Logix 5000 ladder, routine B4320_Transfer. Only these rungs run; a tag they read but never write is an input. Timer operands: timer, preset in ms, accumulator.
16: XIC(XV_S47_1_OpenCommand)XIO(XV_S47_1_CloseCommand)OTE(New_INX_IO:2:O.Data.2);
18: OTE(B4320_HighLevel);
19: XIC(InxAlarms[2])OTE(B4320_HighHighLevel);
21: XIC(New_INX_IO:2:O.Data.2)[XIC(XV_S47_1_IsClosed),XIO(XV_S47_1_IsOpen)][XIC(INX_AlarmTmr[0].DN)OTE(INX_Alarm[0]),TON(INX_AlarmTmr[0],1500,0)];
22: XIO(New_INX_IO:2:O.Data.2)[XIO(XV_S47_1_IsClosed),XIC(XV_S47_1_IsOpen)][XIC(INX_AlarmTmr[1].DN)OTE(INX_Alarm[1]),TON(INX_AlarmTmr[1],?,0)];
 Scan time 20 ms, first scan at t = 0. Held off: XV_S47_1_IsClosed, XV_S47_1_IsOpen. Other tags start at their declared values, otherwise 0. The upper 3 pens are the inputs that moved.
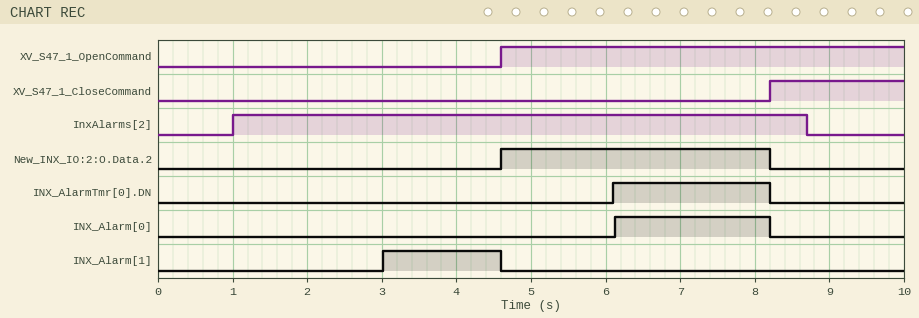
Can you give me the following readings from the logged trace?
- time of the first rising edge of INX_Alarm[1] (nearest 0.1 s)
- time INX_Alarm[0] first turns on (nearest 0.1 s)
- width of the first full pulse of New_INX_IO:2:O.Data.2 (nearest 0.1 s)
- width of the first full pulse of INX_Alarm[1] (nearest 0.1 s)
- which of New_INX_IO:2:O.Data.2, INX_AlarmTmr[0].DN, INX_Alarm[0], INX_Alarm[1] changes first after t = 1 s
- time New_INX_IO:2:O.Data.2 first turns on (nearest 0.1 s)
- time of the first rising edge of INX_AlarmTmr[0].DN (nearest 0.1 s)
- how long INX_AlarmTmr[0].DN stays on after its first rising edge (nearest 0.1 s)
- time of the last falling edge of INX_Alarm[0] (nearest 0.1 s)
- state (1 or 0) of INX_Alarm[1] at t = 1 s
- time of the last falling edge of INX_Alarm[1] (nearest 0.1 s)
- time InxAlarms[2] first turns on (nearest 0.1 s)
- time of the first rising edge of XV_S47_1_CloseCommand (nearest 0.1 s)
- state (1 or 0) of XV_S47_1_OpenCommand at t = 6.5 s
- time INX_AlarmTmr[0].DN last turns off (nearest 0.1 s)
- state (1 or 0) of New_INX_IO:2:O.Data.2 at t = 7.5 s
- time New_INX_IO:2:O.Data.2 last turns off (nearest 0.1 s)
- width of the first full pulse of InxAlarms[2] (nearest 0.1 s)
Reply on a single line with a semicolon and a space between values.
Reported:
3.0 s; 6.1 s; 3.6 s; 1.6 s; INX_Alarm[1]; 4.6 s; 6.1 s; 2.1 s; 8.2 s; 0; 4.6 s; 1.0 s; 8.2 s; 1; 8.2 s; 1; 8.2 s; 7.7 s
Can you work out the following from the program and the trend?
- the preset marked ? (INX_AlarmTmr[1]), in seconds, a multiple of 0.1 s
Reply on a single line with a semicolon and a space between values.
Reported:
3.0 s
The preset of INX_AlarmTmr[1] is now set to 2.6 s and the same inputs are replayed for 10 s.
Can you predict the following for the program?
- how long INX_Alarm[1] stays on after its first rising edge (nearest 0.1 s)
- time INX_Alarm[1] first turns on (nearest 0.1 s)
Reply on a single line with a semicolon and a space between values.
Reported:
2.0 s; 2.6 s
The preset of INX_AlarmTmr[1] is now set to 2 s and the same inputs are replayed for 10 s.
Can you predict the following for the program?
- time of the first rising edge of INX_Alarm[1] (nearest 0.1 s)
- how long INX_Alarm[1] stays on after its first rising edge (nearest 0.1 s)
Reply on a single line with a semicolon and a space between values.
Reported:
2.0 s; 2.6 s
